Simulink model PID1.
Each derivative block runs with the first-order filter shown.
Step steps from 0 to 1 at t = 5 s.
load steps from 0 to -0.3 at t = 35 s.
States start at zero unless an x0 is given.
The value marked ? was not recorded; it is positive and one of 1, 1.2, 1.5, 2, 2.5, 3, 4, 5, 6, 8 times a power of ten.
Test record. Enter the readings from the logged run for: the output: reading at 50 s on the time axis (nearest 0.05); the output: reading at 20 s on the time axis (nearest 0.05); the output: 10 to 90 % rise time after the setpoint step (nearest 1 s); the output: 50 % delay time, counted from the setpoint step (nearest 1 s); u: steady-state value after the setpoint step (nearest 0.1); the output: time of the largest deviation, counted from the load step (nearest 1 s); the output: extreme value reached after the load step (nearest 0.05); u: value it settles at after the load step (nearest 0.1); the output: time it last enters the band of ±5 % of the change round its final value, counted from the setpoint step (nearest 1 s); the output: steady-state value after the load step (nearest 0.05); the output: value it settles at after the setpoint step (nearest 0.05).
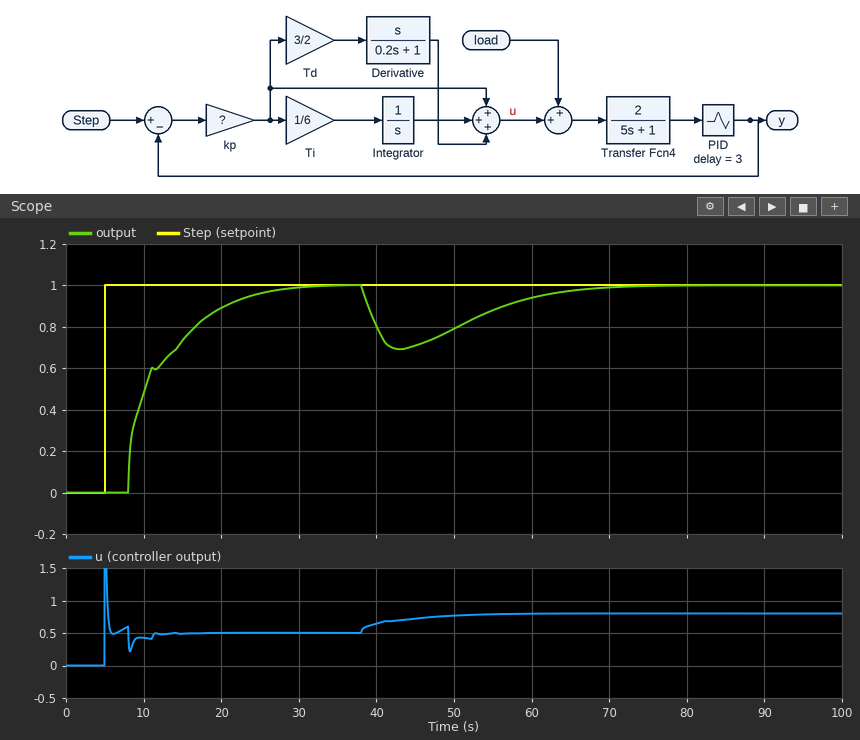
0.80
0.90
12 s
5 s
0.5
8 s
0.70
0.8
19 s
1.00
1.00
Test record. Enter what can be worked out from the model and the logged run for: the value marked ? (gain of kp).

0.4
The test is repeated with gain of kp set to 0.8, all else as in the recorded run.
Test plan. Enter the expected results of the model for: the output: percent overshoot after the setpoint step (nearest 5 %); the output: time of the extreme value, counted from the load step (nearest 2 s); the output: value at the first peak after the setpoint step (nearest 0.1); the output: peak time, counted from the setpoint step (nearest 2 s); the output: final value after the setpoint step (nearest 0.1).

20 %
6 s
1.2
6 s
1.0
